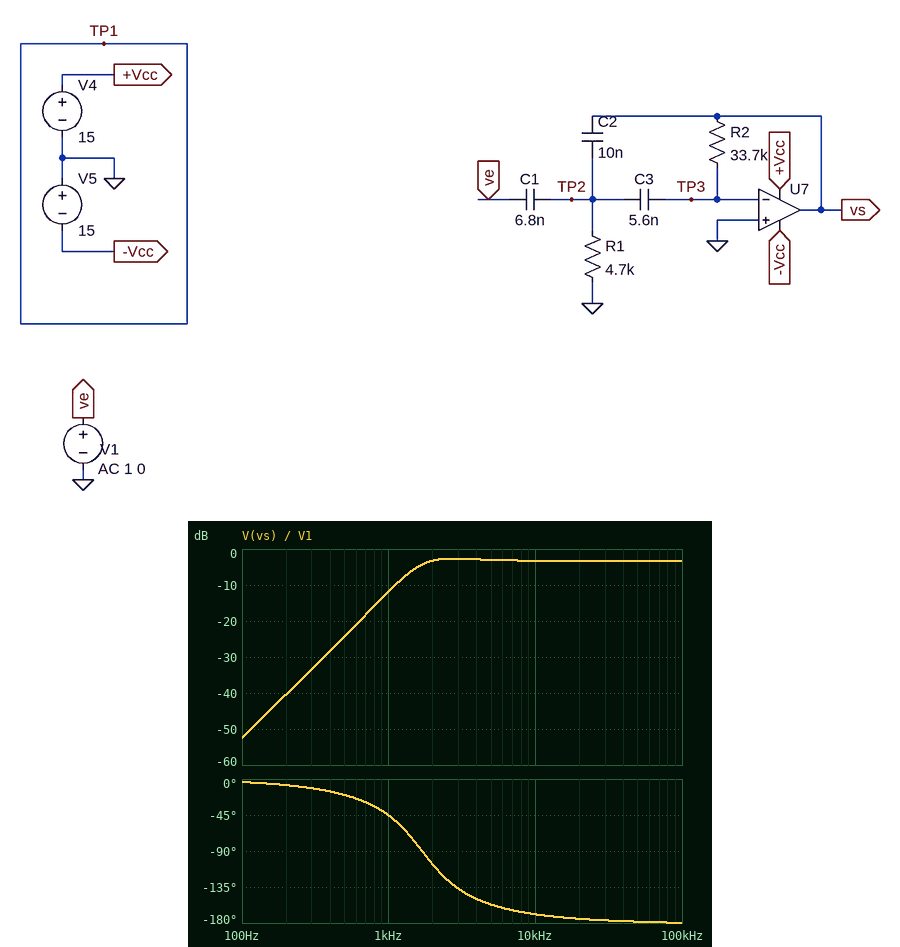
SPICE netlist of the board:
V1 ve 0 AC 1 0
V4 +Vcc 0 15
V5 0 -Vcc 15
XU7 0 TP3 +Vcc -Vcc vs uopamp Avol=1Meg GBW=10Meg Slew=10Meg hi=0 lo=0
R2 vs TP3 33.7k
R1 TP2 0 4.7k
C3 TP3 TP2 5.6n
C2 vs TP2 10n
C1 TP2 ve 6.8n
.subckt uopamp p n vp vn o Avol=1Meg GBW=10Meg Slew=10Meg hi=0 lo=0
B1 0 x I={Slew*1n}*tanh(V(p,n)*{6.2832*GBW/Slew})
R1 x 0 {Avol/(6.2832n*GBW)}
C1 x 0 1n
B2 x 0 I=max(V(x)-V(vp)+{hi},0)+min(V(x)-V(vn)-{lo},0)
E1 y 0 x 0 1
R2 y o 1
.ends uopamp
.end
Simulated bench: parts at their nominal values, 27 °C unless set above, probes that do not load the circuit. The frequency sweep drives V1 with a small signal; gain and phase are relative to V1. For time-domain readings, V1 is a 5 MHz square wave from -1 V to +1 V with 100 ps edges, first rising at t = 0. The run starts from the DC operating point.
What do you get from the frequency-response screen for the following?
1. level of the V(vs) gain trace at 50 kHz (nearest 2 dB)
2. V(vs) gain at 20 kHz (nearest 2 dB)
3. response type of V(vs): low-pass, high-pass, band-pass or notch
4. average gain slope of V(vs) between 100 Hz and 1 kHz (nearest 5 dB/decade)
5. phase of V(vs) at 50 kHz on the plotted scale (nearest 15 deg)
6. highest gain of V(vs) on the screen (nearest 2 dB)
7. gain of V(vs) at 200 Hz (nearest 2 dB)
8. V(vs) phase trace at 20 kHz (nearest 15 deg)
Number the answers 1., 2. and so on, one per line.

1. -4 dB
2. -4 dB
3. high-pass
4. 40 dB/decade
5. -180 deg
6. -2 dB
7. -40 dB
8. -180 deg
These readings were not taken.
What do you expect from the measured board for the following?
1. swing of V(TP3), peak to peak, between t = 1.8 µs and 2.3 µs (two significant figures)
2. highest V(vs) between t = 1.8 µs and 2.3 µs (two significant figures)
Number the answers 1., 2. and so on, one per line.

1. 3.7 V
2. 1.8 V
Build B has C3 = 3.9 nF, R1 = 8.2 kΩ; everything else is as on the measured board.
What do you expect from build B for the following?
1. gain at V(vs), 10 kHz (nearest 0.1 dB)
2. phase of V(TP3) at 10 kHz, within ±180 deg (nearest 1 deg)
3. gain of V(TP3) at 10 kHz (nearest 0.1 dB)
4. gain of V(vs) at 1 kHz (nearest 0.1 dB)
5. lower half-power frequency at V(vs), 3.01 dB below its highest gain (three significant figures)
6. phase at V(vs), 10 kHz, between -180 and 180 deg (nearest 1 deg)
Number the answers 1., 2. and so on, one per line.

1. -3.4 dB
2. 104 deg
3. -63.4 dB
4. -12.4 dB
5. 1.81 kHz
6. -166 deg
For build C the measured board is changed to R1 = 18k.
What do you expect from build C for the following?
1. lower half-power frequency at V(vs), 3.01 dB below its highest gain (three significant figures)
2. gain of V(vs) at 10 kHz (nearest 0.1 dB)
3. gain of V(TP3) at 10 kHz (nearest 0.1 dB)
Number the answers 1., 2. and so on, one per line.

1. 1.52 kHz
2. -3.4 dB
3. -63.4 dB
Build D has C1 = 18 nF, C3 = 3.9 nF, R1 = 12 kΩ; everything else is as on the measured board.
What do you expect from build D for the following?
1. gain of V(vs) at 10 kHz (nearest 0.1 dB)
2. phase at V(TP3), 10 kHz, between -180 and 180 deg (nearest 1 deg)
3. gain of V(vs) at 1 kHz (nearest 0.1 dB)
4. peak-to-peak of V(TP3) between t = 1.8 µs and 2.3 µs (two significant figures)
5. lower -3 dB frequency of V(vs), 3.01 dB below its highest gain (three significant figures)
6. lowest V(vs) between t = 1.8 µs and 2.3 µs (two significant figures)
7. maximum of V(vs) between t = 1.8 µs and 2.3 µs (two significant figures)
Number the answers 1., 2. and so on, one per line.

1. 4.6 dB
2. 111 deg
3. -6.7 dB
4. 3.0 V
5. 3.45 kHz
6. -3.5 V
7. 1.4 V
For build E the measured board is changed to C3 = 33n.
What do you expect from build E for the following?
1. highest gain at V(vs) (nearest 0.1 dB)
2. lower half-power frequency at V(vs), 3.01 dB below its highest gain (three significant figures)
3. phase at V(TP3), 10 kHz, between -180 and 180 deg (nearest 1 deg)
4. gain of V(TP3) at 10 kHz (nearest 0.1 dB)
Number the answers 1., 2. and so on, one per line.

1. -2.2 dB
2. 598 Hz
3. 94 deg
4. -63.3 dB
